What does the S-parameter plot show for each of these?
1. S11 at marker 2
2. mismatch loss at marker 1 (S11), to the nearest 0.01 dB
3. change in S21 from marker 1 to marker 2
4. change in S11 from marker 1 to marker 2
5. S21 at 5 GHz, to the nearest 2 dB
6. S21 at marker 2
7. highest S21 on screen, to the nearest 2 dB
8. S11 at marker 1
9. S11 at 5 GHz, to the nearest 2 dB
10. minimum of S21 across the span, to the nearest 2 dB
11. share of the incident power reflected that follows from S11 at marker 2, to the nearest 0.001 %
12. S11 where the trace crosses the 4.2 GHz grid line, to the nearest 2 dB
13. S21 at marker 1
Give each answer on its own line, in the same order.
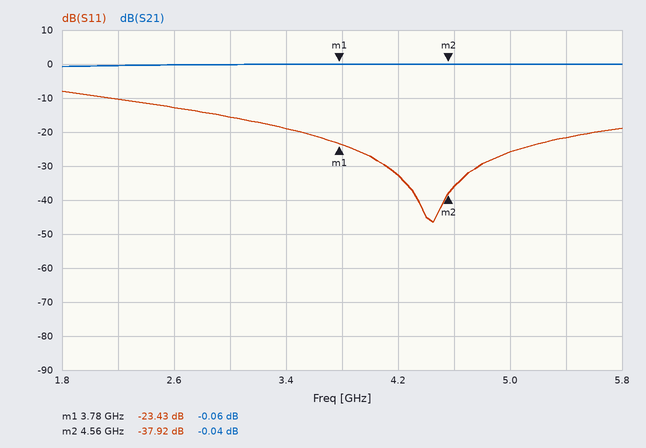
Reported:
-37.92 dB
0.02 dB
0.02 dB
-14.49 dB
0 dB
-0.04 dB
0 dB
-23.43 dB
-26 dB
0 dB
0.016 %
-32 dB
-0.06 dB
